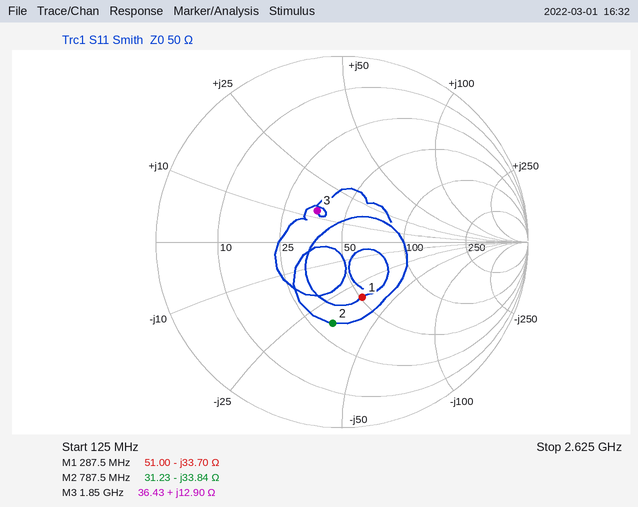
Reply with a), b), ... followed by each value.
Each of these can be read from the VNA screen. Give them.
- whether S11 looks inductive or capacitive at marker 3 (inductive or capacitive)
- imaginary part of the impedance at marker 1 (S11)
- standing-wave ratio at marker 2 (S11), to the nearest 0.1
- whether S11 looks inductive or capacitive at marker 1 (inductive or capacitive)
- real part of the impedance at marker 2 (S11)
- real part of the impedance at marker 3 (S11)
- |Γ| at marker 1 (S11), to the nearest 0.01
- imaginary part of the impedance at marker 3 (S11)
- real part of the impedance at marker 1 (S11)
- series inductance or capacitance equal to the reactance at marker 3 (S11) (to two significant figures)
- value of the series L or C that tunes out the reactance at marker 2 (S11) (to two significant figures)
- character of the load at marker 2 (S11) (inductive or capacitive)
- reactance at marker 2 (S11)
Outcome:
a) inductive
b) -33.70 Ω
c) 2.6
d) capacitive
e) 31.23 Ω
f) 36.43 Ω
g) 0.32
h) +12.90 Ω
i) 51.00 Ω
j) 1.1 nH
k) 6.8 nH
l) capacitive
m) -33.84 Ω
